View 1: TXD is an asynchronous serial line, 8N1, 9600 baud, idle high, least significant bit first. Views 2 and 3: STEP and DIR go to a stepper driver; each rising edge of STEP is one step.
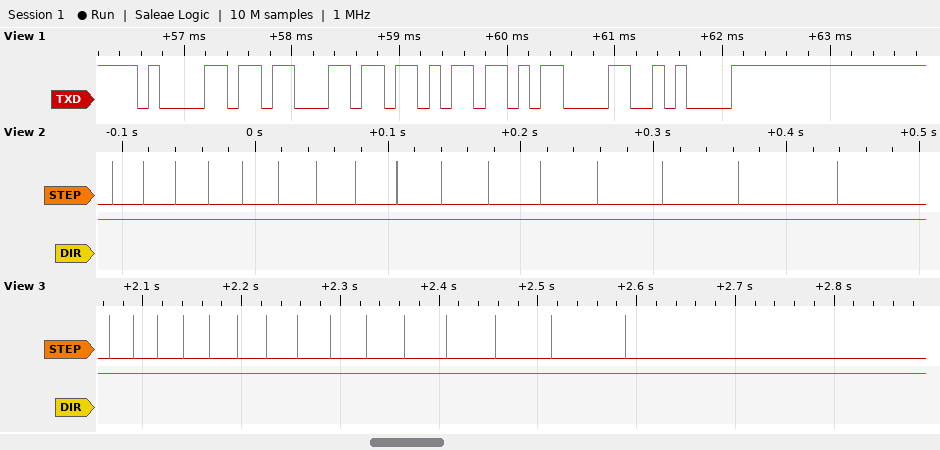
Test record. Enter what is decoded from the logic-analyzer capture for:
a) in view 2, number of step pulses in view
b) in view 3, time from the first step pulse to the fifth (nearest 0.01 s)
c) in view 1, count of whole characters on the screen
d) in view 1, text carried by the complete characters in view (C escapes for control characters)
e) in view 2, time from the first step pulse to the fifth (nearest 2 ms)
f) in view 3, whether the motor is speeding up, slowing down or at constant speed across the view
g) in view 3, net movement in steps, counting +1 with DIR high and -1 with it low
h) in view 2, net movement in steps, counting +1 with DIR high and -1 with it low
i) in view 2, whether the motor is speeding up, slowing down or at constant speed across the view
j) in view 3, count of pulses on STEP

16
0.10 s
5
"ack\r\n"
98 ms
slowing down
+15
+16
slowing down
15
